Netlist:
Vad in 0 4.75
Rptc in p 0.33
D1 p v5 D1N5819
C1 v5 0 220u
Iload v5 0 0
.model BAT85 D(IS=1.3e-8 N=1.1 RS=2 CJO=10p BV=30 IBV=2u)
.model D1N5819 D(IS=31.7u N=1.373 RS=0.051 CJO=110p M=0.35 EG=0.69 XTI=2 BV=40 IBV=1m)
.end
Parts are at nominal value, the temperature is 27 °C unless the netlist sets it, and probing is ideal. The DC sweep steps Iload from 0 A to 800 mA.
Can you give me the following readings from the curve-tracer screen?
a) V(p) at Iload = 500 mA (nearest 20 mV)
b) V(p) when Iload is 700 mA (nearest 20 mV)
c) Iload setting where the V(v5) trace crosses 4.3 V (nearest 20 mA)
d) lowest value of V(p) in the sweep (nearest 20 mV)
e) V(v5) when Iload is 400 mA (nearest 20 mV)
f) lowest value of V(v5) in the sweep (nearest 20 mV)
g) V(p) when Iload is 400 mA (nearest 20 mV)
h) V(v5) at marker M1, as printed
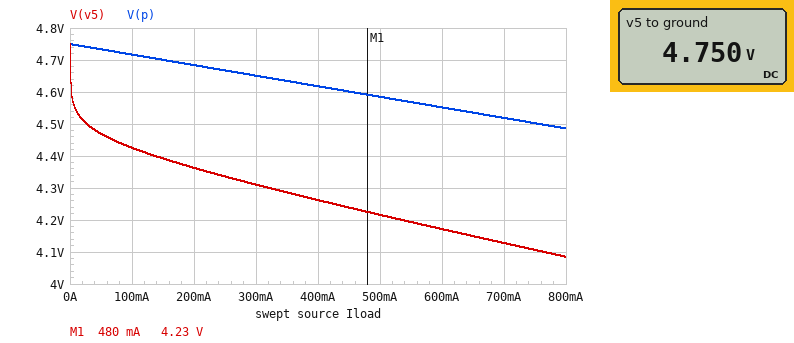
4.58 V
4.52 V
320 mA
4.48 V
4.26 V
4.08 V
4.62 V
4.23 V
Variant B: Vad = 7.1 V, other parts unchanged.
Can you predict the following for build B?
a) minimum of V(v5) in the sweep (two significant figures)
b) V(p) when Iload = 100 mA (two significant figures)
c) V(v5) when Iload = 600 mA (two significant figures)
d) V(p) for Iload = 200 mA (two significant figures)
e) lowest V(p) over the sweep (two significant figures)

6.4 V
7.1 V
6.5 V
7.0 V
6.8 V
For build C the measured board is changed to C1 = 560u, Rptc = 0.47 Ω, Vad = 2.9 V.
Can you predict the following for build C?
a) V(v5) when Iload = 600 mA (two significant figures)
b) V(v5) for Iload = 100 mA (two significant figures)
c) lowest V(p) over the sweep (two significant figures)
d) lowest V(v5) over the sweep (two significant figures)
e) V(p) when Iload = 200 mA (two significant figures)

2.2 V
2.6 V
2.5 V
2.1 V
2.8 V
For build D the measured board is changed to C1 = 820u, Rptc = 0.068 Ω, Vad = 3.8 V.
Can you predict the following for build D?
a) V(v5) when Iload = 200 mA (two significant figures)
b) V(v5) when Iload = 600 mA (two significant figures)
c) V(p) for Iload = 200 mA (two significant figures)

3.5 V
3.4 V
3.8 V
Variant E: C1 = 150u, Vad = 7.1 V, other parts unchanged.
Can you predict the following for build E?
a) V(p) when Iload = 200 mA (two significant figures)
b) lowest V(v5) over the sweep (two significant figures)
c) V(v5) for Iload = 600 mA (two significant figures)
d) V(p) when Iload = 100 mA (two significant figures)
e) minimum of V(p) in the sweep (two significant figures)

7.0 V
6.4 V
6.5 V
7.1 V
6.8 V
